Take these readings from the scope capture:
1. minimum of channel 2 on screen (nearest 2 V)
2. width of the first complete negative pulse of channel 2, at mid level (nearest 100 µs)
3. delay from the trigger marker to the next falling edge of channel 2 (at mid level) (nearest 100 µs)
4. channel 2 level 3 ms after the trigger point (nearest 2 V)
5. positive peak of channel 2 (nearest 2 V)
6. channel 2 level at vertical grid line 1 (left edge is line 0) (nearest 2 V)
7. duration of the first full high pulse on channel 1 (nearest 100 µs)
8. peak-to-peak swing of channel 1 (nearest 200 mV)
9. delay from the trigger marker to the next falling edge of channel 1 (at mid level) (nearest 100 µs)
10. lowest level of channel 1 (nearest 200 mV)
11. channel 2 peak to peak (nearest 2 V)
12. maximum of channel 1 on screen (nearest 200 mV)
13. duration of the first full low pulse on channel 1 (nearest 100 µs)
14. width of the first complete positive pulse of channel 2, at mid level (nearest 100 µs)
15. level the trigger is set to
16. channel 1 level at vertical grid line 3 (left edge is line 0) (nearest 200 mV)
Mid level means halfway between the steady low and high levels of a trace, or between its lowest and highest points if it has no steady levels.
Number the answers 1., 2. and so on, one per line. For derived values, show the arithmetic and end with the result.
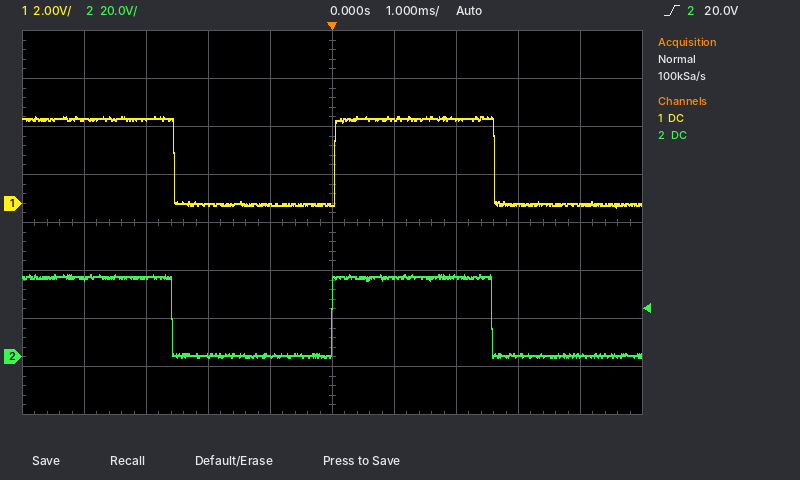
1. 0 V
2. 2.6 ms
3. 2.6 ms
4. 0 V
5. 34 V
6. 32 V
7. 2.6 ms
8. 3.6 V − (-200 mV) = 3.8 V
9. 2.6 ms
10. -200 mV
11. 34 V − (0 V) = 34 V
12. 3.6 V
13. 2.6 ms
14. 2.6 ms
15. 20.0 V
16. 0.0 V
